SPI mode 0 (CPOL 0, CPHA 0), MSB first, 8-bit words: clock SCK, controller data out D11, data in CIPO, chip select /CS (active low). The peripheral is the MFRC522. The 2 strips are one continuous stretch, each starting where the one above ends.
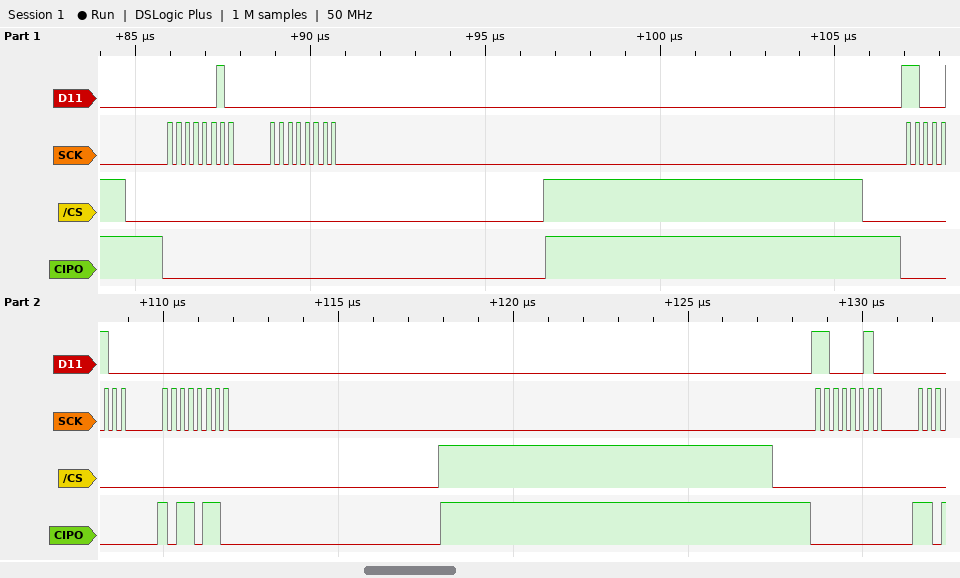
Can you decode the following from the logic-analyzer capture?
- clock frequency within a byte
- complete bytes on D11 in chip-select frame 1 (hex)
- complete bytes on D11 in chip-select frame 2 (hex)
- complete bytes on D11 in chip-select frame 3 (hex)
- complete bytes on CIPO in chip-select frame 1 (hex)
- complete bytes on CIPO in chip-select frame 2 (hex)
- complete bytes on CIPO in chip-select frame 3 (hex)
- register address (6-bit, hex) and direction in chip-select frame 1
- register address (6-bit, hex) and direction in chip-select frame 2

4 MHz
02 00
C4 00
C2
00 00
00 B6
00
0x01 write
0x22 read
